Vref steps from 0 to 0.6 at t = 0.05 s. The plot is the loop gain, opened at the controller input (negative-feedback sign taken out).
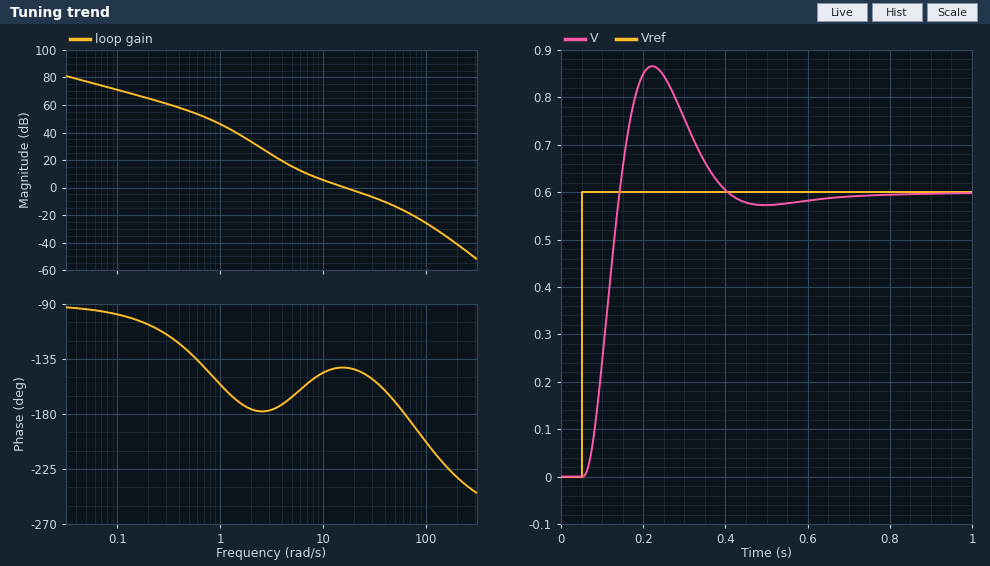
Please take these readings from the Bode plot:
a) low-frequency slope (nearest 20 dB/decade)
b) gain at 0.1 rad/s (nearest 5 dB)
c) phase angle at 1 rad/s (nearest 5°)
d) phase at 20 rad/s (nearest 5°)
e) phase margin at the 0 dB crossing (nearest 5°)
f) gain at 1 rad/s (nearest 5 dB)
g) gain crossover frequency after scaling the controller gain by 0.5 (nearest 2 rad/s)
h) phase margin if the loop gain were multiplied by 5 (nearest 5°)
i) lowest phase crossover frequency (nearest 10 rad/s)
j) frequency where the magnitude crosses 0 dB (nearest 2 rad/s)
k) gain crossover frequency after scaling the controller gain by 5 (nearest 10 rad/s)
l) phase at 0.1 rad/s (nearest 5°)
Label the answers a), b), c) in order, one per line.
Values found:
a) -20 dB/decade
b) 70 dB
c) -155°
d) -145°
e) 40°
f) 45 dB
g) 10 rad/s
h) 10°
i) 60 rad/s
j) 16 rad/s
k) 50 rad/s
l) -100°
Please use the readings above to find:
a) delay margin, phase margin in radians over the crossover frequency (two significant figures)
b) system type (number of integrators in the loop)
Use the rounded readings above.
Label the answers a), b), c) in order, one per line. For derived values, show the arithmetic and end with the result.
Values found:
a) 40 × π / 180 / 16 = 0.044 s
b) 1
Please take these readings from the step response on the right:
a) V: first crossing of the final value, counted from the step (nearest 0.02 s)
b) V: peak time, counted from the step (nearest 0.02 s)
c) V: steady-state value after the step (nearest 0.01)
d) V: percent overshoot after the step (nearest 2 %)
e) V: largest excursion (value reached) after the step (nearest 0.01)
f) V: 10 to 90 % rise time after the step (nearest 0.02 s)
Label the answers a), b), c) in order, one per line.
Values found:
a) 0.10 s
b) 0.18 s
c) 0.60
d) 44 %
e) 0.87
f) 0.06 s
